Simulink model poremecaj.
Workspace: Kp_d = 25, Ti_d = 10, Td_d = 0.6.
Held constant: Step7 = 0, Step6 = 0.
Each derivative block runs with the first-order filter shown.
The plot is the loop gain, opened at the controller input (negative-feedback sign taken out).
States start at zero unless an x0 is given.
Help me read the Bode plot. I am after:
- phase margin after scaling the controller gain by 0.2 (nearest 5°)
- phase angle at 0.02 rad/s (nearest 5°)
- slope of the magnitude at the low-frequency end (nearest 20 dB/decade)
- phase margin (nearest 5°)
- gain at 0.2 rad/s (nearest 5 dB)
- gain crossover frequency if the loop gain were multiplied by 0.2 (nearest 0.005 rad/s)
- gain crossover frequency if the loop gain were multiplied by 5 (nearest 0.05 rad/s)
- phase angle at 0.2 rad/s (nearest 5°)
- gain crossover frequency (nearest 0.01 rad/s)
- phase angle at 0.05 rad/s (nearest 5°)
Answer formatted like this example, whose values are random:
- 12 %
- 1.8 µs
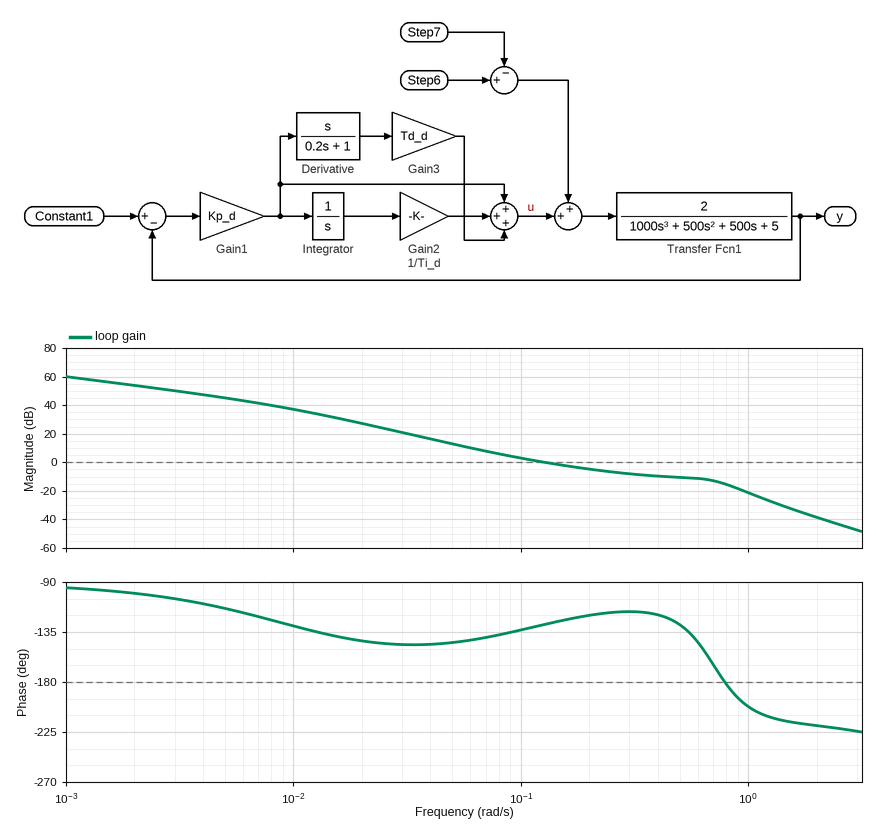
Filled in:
- 35°
- -145°
- -20 dB/decade
- 50°
- -5 dB
- 0.045 rad/s
- 0.75 rad/s
- -120°
- 0.13 rad/s
- -145°
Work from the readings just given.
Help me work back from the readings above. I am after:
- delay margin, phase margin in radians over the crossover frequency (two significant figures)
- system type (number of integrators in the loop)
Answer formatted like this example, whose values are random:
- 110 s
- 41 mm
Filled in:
- 6.7 s
- 1
